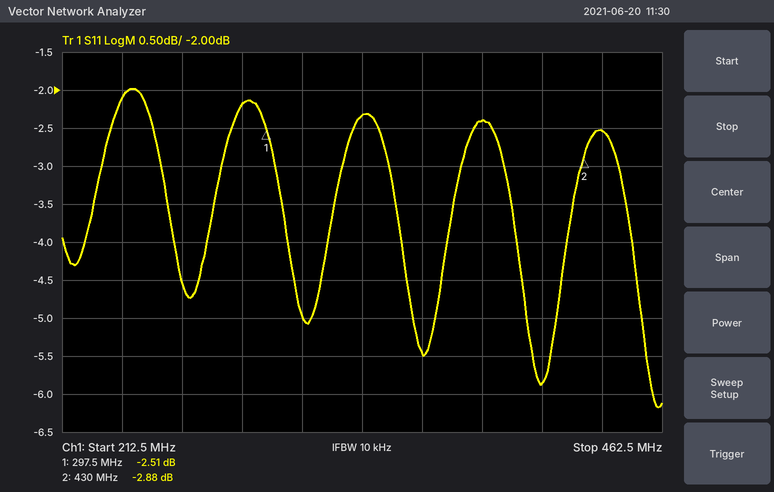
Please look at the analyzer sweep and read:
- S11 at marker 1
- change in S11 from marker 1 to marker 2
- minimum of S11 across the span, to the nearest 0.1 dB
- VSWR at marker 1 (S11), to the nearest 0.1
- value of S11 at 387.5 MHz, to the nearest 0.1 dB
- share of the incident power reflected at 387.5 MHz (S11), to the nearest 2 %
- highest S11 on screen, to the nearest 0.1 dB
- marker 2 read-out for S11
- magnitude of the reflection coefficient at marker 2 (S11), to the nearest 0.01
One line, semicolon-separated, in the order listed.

-2.51 dB; -0.37 dB; -6.2 dB; 7.0; -2.4 dB; 58 %; -2.0 dB; -2.88 dB; 0.72
